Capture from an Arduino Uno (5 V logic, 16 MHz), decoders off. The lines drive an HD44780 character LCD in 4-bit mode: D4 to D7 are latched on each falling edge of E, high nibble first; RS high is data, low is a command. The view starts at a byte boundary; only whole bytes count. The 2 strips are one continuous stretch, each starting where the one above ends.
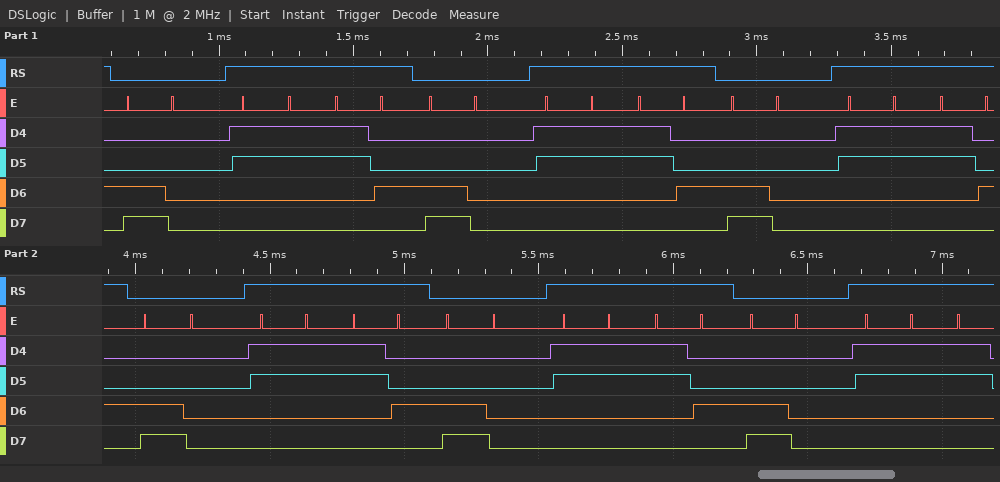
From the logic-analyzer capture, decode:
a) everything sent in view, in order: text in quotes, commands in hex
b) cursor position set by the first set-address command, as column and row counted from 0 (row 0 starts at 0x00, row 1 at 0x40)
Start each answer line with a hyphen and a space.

- 0xC0 "34" 0xC0 "34" 0xC0 "34" 0xC0 "34" 0xC0 "34" 0xC0 "3"
- column 0, row 1
